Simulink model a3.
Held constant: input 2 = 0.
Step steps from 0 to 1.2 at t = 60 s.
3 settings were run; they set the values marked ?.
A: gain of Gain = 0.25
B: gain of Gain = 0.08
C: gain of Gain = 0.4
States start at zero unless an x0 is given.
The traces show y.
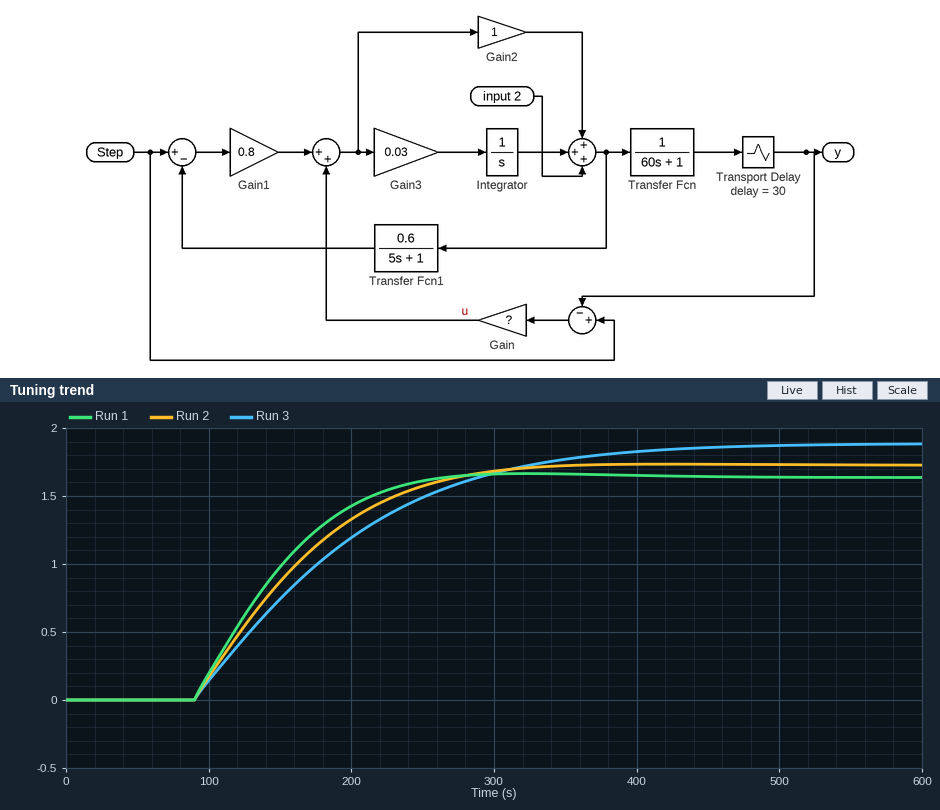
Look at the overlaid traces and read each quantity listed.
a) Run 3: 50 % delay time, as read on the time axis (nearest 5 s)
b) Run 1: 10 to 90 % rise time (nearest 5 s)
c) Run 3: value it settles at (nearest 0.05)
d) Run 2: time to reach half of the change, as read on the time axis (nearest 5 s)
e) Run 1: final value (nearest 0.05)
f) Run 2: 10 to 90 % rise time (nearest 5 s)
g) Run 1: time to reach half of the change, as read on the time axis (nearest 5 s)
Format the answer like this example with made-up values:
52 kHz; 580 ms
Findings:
170 s; 110 s; 1.90; 150 s; 1.65; 145 s; 140 s
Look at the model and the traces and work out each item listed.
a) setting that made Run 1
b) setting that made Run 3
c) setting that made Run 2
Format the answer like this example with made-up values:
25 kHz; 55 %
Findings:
C; B; A
